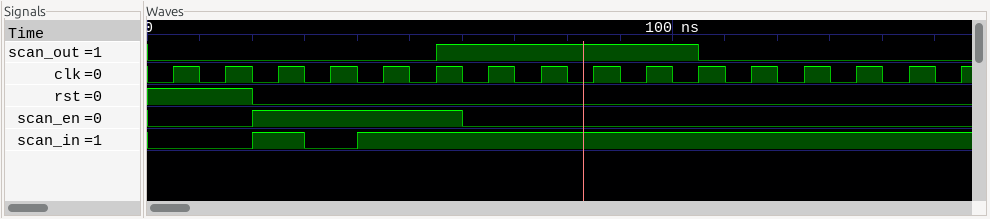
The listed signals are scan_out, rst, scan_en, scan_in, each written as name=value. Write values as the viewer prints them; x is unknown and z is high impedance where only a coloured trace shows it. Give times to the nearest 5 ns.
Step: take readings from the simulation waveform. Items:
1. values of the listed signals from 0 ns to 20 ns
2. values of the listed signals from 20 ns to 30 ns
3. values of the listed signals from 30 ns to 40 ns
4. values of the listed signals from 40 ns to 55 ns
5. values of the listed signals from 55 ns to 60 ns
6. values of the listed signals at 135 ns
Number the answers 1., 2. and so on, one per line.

1. scan_out=0, rst=1, scan_en=0, scan_in=0
2. scan_out=0, rst=0, scan_en=1, scan_in=1
3. scan_out=0, rst=0, scan_en=1, scan_in=0
4. scan_out=0, rst=0, scan_en=1, scan_in=1
5. scan_out=1, rst=0, scan_en=1, scan_in=1
6. scan_out=0, rst=0, scan_en=0, scan_in=1
